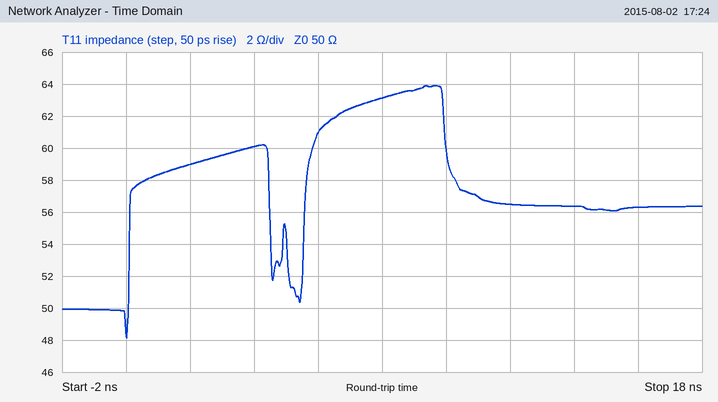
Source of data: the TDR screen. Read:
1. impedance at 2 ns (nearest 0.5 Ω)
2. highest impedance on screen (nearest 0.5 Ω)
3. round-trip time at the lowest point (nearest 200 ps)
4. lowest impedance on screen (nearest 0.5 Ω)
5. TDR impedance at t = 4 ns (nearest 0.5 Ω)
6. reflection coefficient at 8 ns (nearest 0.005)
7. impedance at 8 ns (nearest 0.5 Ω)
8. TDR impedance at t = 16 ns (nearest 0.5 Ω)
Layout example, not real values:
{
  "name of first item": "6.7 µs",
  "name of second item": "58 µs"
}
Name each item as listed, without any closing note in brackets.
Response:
{
  "impedance at 2 ns": "59.0 Ω",
  "highest impedance on screen": "64.0 Ω",
  "round-trip time at the lowest point": "0.0 ns",
  "lowest impedance on screen": "48.0 Ω",
  "TDR impedance at t = 4 ns": "60.0 Ω",
  "reflection coefficient at 8 ns": "+0.115",
  "impedance at 8 ns": "63.0 Ω",
  "TDR impedance at t = 16 ns": "56.5 Ω"
}
